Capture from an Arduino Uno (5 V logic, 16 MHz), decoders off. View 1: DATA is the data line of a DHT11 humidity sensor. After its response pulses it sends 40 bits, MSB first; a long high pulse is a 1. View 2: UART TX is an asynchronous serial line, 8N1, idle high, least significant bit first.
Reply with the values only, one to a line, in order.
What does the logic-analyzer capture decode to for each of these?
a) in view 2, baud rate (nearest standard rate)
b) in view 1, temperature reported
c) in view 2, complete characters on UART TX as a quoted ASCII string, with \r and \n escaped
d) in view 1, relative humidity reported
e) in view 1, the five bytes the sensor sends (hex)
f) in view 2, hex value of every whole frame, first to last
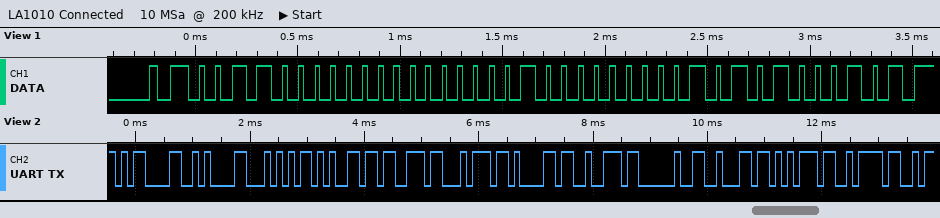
9600 baud
16.5 °C
"\r\nTestar buz"
48 %
30 00 10 05 45
0x0D 0x0A 0x54 0x65 0x73 0x74 0x61 0x72 0x20 0x62 0x75 0x7A
